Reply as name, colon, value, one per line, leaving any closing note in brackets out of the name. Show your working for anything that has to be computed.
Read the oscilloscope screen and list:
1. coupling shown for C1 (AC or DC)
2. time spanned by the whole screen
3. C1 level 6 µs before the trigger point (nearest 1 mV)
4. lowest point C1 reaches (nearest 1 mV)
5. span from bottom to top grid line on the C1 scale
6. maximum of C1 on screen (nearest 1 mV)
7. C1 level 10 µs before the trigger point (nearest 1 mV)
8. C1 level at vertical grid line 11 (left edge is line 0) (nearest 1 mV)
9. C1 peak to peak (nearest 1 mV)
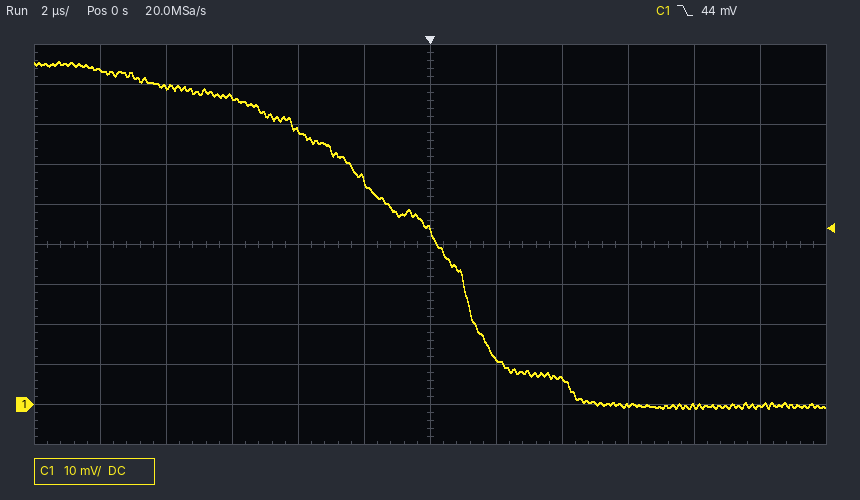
coupling shown for C1: DC
time spanned by the whole screen: 24 µs
C1 level 6 µs before the trigger point: 77 mV
lowest point C1 reaches: -1 mV
span from bottom to top grid line on the C1 scale: 100 mV
maximum of C1 on screen: 86 mV
C1 level 10 µs before the trigger point: 84 mV
C1 level at vertical grid line 11 (left edge is line 0): 0 mV
C1 peak to peak: 86 mV − (-1 mV) = 87 mV
